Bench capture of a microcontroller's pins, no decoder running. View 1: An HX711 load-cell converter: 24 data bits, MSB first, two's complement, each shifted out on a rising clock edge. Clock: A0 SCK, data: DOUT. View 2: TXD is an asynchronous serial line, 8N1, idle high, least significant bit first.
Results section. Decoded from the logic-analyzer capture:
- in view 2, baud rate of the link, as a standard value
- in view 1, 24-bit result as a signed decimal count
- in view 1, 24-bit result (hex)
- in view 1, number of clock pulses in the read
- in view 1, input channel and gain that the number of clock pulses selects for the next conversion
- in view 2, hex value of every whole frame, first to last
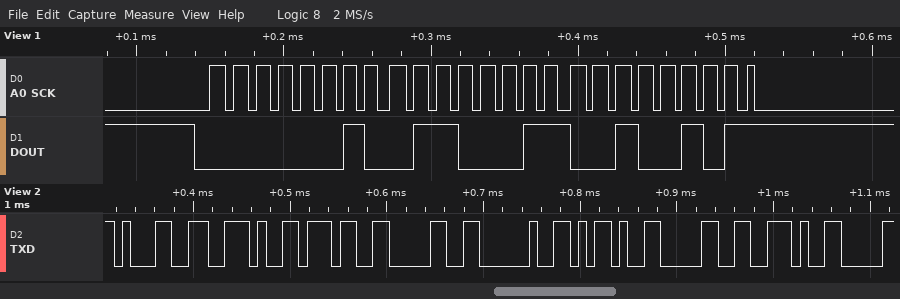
115200 baud
156453
0x026325
25
channel A, gain 128
31 2E 37 30 20 2D 30 2E
